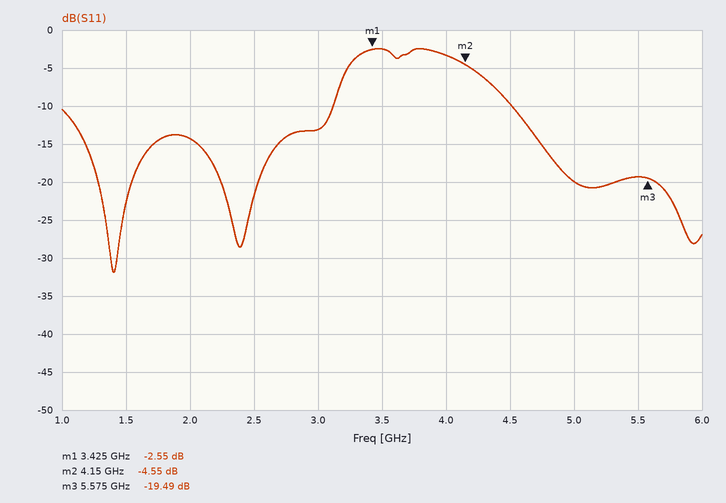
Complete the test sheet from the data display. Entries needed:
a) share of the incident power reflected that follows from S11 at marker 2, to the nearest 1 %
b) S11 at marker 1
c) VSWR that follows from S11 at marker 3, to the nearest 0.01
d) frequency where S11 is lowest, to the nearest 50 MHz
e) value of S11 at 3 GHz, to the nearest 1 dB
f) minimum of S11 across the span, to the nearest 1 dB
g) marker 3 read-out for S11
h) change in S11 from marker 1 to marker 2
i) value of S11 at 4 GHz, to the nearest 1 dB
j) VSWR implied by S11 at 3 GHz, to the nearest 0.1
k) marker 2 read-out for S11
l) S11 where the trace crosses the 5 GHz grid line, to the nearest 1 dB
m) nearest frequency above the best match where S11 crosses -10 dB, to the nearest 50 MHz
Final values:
35 %
-2.55 dB
1.24
1.40 GHz
-13 dB
-32 dB
-19.49 dB
-2.00 dB
-3 dB
1.6
-4.55 dB
-20 dB
3.10 GHz
